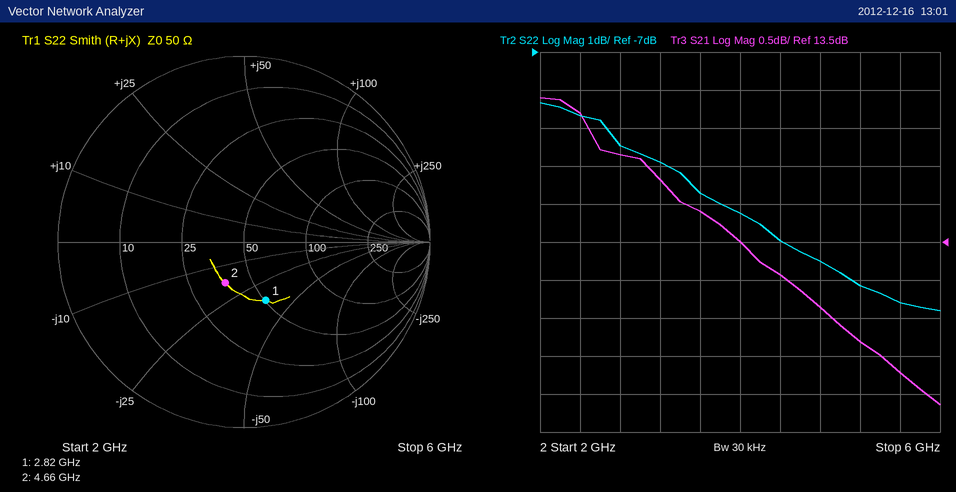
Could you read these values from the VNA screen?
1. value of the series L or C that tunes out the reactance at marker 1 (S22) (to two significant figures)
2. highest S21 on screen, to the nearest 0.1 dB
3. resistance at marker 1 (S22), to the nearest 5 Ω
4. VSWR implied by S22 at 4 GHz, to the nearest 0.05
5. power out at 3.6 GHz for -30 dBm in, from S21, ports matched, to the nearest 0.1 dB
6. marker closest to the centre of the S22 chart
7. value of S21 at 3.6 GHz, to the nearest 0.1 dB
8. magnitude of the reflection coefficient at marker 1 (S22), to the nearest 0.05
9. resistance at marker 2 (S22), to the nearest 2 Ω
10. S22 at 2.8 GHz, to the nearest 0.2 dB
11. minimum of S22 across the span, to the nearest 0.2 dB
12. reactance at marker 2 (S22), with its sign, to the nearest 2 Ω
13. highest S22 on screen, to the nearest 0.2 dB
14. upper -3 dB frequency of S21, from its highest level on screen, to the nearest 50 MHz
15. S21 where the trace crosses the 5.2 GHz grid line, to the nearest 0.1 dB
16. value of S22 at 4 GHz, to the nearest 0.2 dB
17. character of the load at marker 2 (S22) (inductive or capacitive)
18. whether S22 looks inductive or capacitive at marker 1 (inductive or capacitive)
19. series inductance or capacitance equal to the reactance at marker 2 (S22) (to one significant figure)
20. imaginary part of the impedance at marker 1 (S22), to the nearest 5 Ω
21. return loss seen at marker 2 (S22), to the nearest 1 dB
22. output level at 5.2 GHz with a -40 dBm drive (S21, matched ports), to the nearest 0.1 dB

2.0 nH
15.4 dB
50 Ω
1.75
-16.1 dBm
marker 2
13.9 dB
0.35
38 Ω
-9.4 dB
-13.8 dB
-18 Ω
-8.4 dB
5.00 GHz
12.2 dB
-11.2 dB
capacitive
capacitive
2 pF
-35 Ω
12 dB
-27.8 dBm
